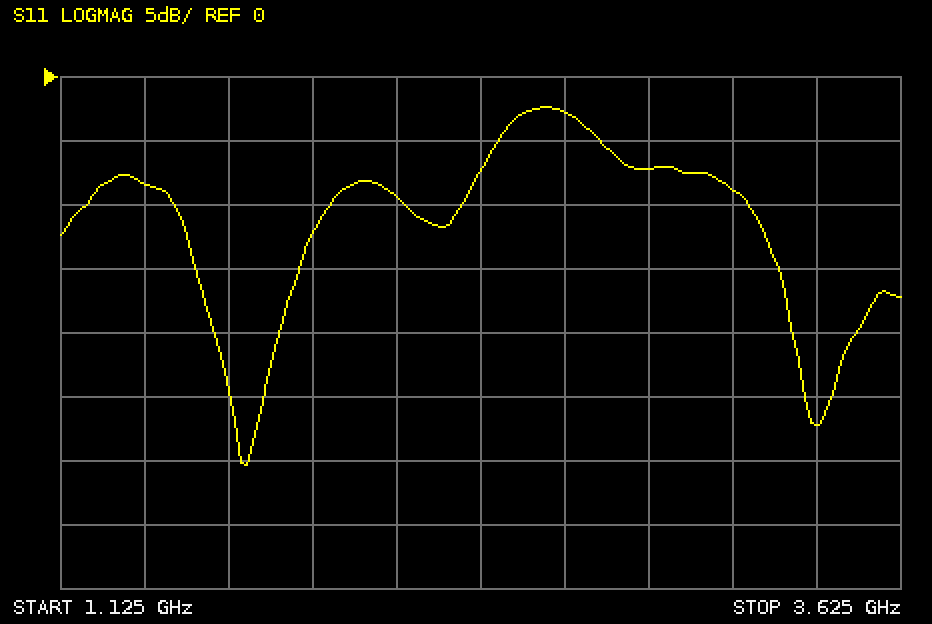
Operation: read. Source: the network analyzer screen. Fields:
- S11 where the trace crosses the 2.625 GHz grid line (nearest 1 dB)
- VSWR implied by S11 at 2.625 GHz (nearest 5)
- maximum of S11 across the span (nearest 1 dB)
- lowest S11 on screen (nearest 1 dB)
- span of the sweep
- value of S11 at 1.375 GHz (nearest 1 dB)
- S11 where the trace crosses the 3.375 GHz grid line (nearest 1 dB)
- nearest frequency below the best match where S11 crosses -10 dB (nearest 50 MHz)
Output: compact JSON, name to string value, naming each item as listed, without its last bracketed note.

{"S11 where the trace crosses the 2.625 GHz grid line": "-3 dB", "VSWR implied by S11 at 2.625 GHz": "5", "maximum of S11 across the span": "-2 dB", "lowest S11 on screen": "-30 dB", "span of the sweep": "2.5 GHz", "value of S11 at 1.375 GHz": "-8 dB", "S11 where the trace crosses the 3.375 GHz grid line": "-27 dB", "nearest frequency below the best match where S11 crosses -10 dB": "1.45 GHz"}
